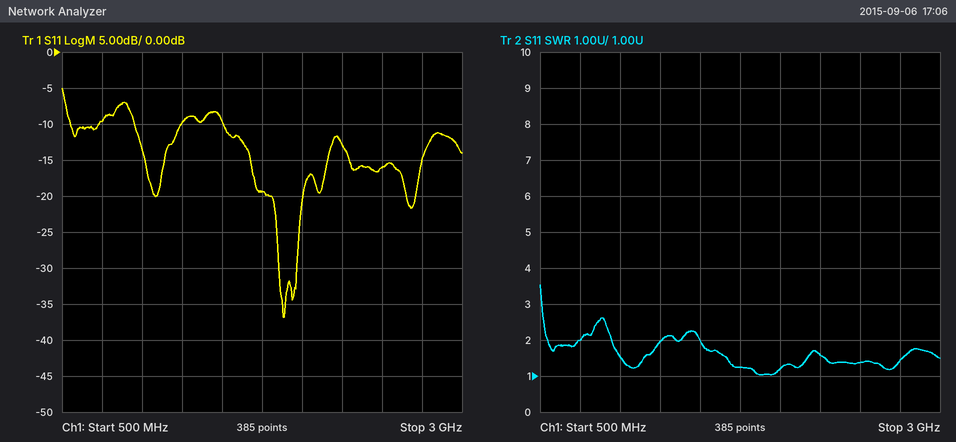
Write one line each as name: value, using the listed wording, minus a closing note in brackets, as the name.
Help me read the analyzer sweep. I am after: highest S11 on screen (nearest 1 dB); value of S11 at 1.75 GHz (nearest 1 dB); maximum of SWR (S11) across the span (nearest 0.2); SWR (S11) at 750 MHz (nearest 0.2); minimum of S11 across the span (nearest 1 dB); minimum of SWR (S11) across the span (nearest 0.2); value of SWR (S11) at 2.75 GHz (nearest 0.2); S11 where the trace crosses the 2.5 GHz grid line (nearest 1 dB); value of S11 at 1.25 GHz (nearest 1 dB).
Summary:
highest S11 on screen: -5 dB
value of S11 at 1.75 GHz: -19 dB
maximum of SWR (S11) across the span: 3.6
SWR (S11) at 750 MHz: 2.0
minimum of S11 across the span: -37 dB
minimum of SWR (S11) across the span: 1.0
value of SWR (S11) at 2.75 GHz: 1.4
S11 where the trace crosses the 2.5 GHz grid line: -16 dB
value of S11 at 1.25 GHz: -10 dB
